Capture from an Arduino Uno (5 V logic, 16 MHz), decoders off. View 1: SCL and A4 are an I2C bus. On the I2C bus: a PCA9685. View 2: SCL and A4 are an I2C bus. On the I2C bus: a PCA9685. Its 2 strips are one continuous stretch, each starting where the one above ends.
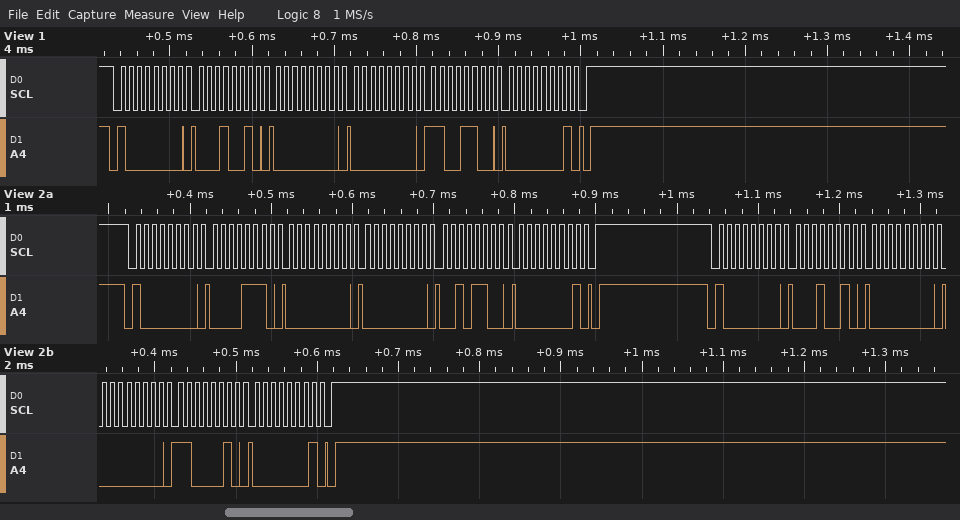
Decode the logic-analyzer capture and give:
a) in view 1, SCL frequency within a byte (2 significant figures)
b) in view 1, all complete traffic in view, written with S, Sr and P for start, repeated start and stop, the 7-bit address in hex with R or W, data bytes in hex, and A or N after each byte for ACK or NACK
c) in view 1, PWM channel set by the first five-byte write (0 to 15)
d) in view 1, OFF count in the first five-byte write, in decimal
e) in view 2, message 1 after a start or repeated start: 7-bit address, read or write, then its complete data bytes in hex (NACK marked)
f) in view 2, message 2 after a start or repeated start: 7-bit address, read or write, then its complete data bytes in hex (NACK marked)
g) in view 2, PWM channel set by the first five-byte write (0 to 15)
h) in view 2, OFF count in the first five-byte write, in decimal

100 kHz
S 40W A 12 A 00 A 00 A CC A 01 A P
3
460
0x40 write: 0E 00 00 2C 01
0x40 write: 12 00 00 C2 01
2
300
